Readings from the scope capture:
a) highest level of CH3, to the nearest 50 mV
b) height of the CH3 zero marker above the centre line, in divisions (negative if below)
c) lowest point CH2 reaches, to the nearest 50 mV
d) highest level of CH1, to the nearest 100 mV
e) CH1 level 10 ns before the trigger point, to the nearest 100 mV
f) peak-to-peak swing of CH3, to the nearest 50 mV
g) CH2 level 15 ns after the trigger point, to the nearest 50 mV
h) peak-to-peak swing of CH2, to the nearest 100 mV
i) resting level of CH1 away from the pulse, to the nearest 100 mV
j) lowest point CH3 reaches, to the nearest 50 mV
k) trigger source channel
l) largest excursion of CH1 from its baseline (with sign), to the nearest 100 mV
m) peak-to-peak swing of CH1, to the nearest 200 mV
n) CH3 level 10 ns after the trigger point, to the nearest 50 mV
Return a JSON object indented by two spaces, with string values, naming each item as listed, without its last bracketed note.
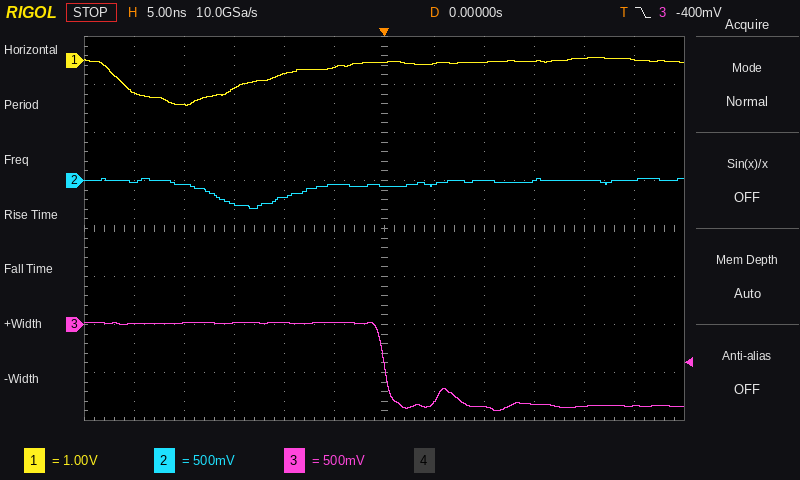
{
  "highest level of CH3, to the nearest 50 mV": "0 mV",
  "height of the CH3 zero marker above the centre line, in divisions": "-2.0 div",
  "lowest point CH2 reaches, to the nearest 50 mV": "-300 mV",
  "highest level of CH1, to the nearest 100 mV": "100 mV",
  "CH1 level 10 ns before the trigger point, to the nearest 100 mV": "-300 mV",
  "peak-to-peak swing of CH3, to the nearest 50 mV": "900 mV",
  "CH2 level 15 ns after the trigger point, to the nearest 50 mV": "0 mV",
  "peak-to-peak swing of CH2, to the nearest 100 mV": "300 mV",
  "resting level of CH1 away from the pulse, to the nearest 100 mV": "0.0 V",
  "lowest point CH3 reaches, to the nearest 50 mV": "-900 mV",
  "trigger source channel": "CH3",
  "largest excursion of CH1 from its baseline (with sign), to the nearest 100 mV": "-900 mV",
  "peak-to-peak swing of CH1, to the nearest 200 mV": "1.0 V",
  "CH3 level 10 ns after the trigger point, to the nearest 50 mV": "-850 mV"
}
